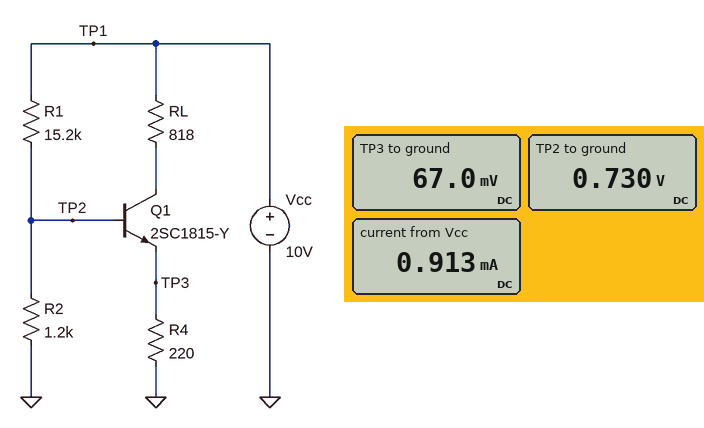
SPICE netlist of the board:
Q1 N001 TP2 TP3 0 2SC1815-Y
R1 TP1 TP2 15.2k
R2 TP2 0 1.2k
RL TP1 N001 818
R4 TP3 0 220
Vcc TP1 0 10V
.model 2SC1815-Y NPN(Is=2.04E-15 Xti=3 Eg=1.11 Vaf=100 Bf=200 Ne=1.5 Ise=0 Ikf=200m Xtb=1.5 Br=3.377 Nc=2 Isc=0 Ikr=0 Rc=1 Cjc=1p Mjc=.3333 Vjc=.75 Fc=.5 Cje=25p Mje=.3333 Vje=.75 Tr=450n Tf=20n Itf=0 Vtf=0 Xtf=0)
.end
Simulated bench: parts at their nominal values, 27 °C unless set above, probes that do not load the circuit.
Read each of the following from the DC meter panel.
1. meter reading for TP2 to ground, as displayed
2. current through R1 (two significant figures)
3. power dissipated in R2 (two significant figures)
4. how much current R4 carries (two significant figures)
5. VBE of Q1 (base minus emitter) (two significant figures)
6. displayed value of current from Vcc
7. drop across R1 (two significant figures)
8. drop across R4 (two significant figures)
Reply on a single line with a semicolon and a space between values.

0.730 V; 610 µA; 440 µW; 300 µA; 660 mV; 0.913 mA; 9.3 V; 67 mV
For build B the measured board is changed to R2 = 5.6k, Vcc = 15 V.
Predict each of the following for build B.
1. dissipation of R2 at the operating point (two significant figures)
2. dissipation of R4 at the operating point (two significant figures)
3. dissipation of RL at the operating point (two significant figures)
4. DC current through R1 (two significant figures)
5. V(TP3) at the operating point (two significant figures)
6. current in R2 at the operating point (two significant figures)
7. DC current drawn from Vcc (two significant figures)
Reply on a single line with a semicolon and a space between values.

2.5 mW; 40 mW; 150 mW; 740 µA; 3.0 V; 670 µA; 14 mA
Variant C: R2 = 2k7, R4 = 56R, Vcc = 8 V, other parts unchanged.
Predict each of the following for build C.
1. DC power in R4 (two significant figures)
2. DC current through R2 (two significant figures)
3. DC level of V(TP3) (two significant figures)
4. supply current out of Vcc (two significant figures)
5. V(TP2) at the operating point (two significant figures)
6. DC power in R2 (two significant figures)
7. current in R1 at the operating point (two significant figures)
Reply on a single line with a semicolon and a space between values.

2.6 mW; 420 µA; 380 mV; 7.2 mA; 1.1 V; 470 µW; 450 µA
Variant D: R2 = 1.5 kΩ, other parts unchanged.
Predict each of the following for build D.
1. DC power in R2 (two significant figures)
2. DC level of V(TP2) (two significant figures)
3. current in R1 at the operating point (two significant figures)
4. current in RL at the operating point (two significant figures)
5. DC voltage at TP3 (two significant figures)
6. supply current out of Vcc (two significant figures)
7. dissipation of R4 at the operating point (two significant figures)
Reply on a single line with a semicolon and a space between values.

530 µW; 890 mV; 600 µA; 910 µA; 200 mV; 1.5 mA; 180 µW
